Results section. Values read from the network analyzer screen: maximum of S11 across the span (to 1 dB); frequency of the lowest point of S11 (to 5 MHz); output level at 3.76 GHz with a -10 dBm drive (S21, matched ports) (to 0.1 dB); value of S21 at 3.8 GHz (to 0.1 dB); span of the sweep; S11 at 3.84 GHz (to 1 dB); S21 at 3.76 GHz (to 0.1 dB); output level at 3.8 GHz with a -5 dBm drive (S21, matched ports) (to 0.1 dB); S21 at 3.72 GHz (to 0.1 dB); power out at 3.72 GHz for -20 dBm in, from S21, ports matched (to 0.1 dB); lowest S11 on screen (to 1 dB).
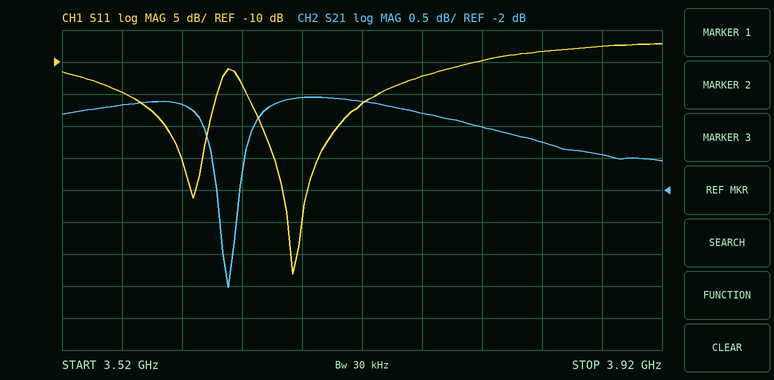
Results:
-7 dB
3.675 GHz
-10.8 dBm
-1.0 dB
400 MHz
-8 dB
-0.8 dB
-6.0 dBm
-0.6 dB
-20.6 dBm
-43 dB
